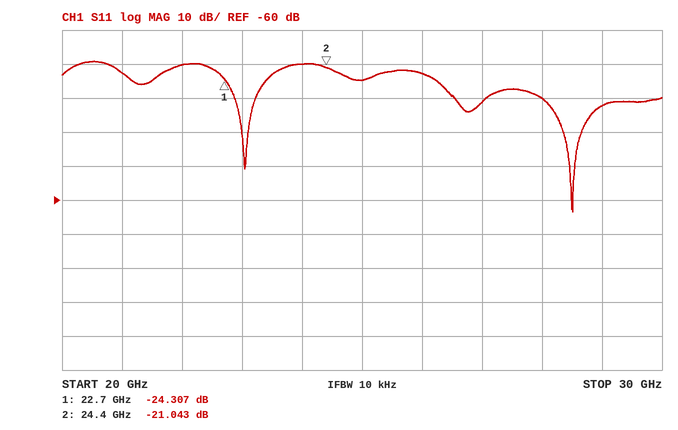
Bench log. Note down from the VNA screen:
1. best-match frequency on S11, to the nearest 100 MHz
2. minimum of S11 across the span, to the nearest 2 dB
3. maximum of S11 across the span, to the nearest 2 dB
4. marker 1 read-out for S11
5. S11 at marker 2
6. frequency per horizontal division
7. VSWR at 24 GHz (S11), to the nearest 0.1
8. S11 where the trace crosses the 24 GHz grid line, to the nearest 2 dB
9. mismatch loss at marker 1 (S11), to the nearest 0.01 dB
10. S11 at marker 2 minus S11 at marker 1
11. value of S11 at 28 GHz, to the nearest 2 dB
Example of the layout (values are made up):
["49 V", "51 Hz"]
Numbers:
["28.5 GHz", "-64 dB", "-20 dB", "-24.307 dB", "-21.043 dB", "1 GHz", "1.2", "-20 dB", "0.02 dB", "3.264 dB", "-30 dB"]
